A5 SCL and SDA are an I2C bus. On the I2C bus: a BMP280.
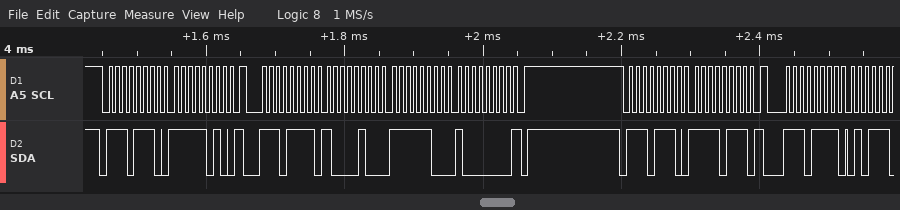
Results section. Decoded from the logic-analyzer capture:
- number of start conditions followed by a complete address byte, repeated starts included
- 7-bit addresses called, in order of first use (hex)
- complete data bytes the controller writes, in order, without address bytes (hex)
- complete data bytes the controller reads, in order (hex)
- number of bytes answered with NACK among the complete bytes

4
0x77
FA F7
84 FC 80
1
